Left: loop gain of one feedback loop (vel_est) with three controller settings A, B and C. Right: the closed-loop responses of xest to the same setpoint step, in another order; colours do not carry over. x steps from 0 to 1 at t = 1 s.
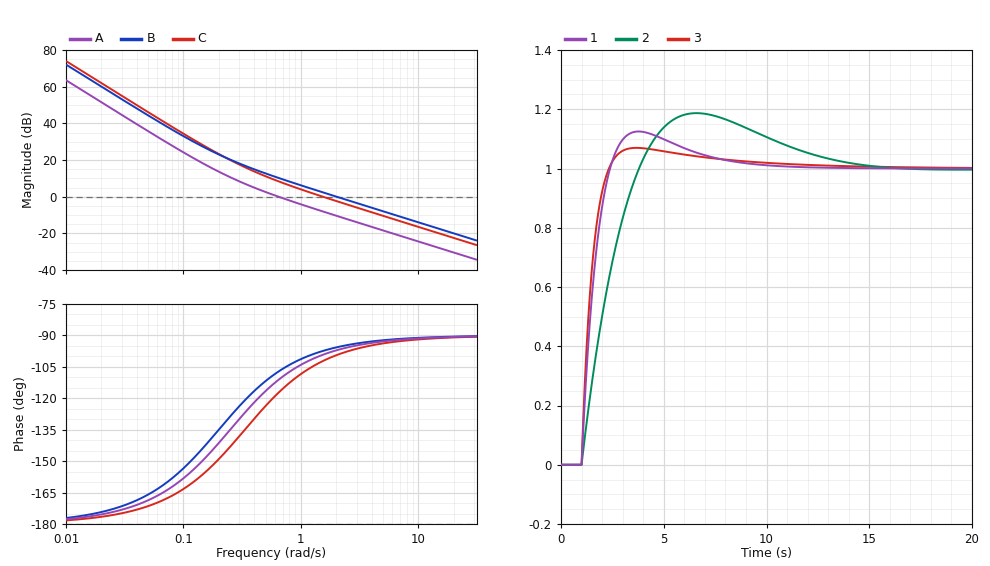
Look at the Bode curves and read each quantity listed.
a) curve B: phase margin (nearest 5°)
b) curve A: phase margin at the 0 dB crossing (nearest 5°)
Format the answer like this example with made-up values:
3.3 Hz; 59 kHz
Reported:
85°; 70°
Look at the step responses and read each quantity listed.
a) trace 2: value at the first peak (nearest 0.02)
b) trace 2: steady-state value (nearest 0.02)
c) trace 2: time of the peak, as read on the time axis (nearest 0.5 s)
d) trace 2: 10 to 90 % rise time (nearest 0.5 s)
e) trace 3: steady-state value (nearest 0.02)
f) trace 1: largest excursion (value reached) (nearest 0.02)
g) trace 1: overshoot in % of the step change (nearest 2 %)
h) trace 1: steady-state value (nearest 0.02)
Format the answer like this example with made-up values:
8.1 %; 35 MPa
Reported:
1.18; 1.00; 6.5 s; 2.0 s; 1.00; 1.12; 12 %; 1.00
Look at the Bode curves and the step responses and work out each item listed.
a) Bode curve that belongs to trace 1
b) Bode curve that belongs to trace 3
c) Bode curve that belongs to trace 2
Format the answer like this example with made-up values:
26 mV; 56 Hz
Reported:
C; B; A
